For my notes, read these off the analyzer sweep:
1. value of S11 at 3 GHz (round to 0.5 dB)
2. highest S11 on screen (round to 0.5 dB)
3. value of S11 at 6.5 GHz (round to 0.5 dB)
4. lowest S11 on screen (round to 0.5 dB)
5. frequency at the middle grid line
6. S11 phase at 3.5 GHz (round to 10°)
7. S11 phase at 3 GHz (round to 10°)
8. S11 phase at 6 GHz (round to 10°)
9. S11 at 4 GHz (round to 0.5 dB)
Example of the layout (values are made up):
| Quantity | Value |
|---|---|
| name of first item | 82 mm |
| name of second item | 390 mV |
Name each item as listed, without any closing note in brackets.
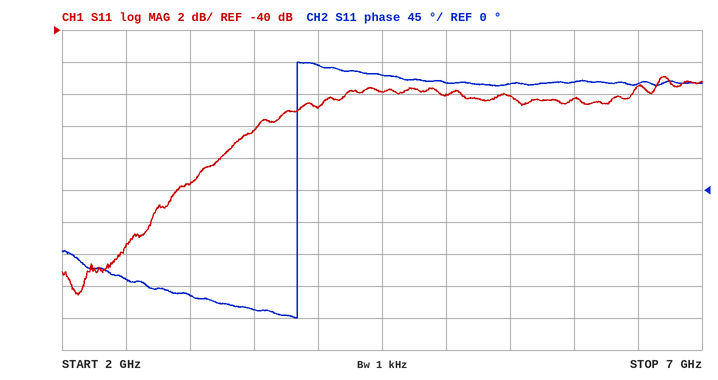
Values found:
| Quantity | Value |
|---|---|
| value of S11 at 3 GHz | -49.5 dB |
| highest S11 on screen | -43.0 dB |
| value of S11 at 6.5 GHz | -43.5 dB |
| lowest S11 on screen | -56.5 dB |
| frequency at the middle grid line | 4.5 GHz |
| S11 phase at 3.5 GHz | -170° |
| S11 phase at 3 GHz | -150° |
| S11 phase at 6 GHz | 150° |
| S11 at 4 GHz | -45.0 dB |
